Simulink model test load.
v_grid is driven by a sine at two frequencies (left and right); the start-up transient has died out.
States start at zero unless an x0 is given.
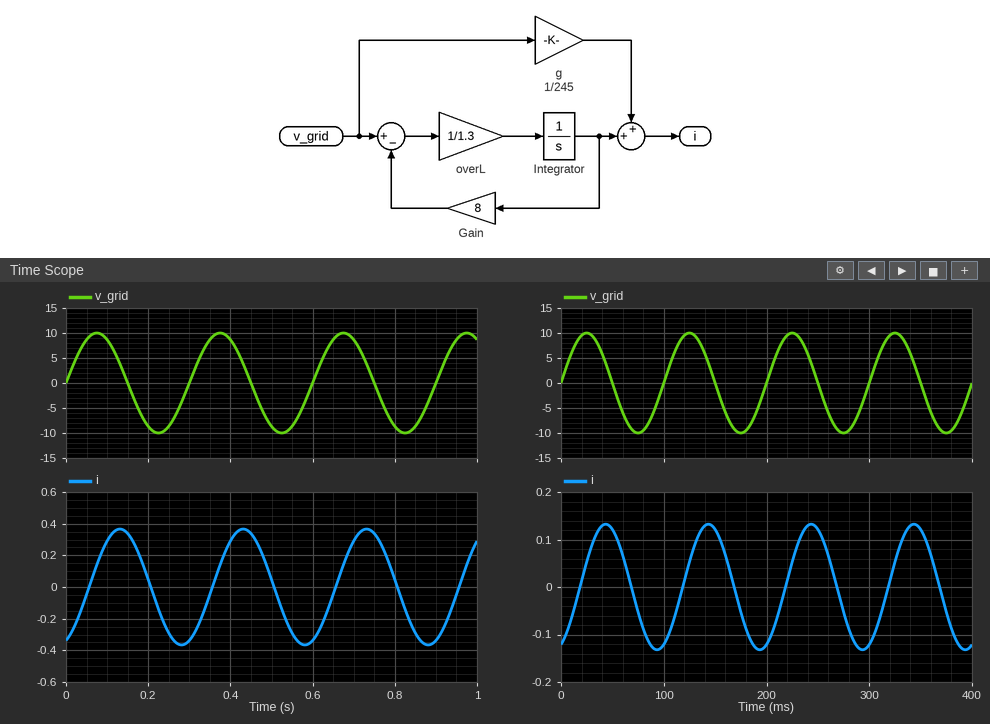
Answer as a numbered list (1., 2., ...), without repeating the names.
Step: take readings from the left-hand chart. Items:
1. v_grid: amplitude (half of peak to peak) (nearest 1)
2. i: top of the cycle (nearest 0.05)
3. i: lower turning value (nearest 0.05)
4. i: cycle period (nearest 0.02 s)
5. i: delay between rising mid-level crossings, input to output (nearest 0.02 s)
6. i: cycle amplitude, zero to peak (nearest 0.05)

1. 10
2. 0.35
3. -0.35
4. 0.30 s
5. 0.06 s
6. 0.35
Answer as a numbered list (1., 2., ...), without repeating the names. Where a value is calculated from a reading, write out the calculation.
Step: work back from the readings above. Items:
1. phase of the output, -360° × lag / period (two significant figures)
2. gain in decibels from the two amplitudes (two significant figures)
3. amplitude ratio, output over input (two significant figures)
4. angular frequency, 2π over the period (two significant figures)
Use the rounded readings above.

1. -360 × 0.06 / 0.3 = -72°
2. 20 log10(0.35 / 10) = -29 dB
3. 0.35 / 10 = 0.035
4. 2π / 0.3 = 21 rad/s
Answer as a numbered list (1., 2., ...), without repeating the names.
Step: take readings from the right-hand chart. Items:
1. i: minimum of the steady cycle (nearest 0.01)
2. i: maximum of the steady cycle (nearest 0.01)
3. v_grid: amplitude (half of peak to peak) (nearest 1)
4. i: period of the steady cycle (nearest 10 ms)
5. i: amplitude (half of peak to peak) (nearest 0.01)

1. -0.13
2. 0.13
3. 10
4. 100 ms
5. 0.13
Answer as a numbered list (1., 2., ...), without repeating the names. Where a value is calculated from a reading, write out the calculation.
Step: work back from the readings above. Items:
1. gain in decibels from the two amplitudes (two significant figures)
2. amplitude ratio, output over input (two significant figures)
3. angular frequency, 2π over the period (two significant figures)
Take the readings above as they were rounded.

1. 20 log10(0.13 / 10) = -38 dB
2. 0.13 / 10 = 0.013
3. 2π / 100 = 0.063 rad/ms
